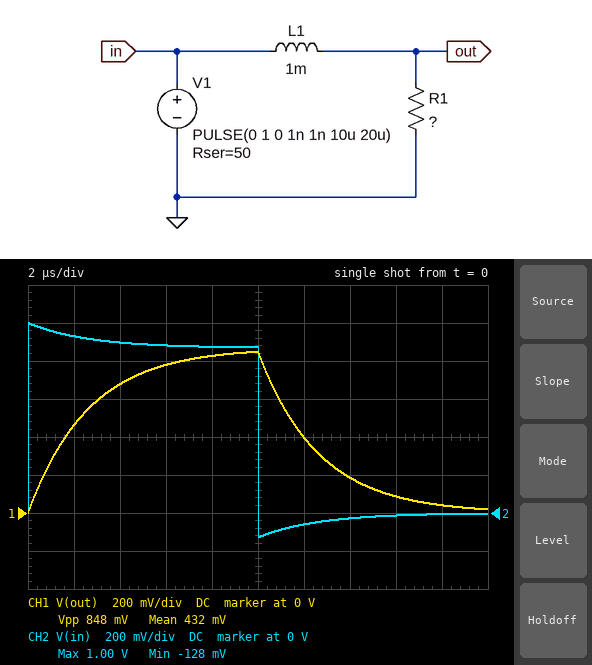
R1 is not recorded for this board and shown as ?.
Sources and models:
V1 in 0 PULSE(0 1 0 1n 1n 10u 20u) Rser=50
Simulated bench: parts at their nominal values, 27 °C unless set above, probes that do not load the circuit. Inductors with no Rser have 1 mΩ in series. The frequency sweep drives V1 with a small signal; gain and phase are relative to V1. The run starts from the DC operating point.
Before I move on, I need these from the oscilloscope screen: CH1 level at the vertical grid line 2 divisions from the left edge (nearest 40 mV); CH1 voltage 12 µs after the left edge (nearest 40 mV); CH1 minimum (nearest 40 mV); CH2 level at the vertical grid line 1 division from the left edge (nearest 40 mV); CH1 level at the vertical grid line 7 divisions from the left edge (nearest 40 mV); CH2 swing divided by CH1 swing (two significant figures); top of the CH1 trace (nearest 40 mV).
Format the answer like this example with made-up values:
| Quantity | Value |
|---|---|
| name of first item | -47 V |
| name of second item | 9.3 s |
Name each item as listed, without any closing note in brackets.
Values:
| Quantity | Value |
|---|---|
| CH1 level at the vertical grid line 2 divisions from the left edge | 680 mV |
| CH1 voltage 12 µs after the left edge | 400 mV |
| CH1 minimum | 0 V |
| CH2 level at the vertical grid line 1 division from the left edge | 920 mV |
| CH1 level at the vertical grid line 7 divisions from the left edge | 200 mV |
| CH2 swing divided by CH1 swing | 1.3 |
| top of the CH1 trace | 840 mV |
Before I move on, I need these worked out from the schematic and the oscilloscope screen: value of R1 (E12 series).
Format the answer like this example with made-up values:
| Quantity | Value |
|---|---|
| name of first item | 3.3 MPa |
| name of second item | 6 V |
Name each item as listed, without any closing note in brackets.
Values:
| Quantity | Value |
|---|---|
| value of R1 | 330 Ω |
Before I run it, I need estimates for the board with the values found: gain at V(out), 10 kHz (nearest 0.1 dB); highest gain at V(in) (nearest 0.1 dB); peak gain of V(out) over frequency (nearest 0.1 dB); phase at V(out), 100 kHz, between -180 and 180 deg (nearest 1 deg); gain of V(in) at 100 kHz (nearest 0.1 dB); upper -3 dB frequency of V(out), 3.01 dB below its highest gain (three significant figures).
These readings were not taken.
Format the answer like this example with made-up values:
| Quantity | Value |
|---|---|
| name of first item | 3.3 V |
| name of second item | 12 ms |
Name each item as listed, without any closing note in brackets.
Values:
| Quantity | Value |
|---|---|
| gain at V(out), 10 kHz | -1.3 dB |
| highest gain at V(in) | 0 dB |
| peak gain of V(out) over frequency | -1.2 dB |
| phase at V(out), 100 kHz, between -180 and 180 deg | -59 deg |
| gain of V(in) at 100 kHz | -0.3 dB |
| upper -3 dB frequency of V(out), 3.01 dB below its highest gain | 60.5 kHz |
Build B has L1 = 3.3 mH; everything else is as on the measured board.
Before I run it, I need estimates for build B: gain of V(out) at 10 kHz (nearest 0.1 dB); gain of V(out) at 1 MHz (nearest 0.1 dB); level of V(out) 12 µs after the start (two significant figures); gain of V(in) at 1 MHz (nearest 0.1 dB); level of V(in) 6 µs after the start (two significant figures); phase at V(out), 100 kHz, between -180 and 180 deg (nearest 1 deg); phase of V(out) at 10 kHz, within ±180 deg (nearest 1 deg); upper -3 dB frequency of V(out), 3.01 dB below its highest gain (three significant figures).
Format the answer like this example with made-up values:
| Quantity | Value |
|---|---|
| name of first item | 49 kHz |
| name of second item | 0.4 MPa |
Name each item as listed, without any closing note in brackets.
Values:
| Quantity | Value |
|---|---|
| gain of V(out) at 10 kHz | -2.4 dB |
| gain of V(out) at 1 MHz | -36.0 dB |
| level of V(out) 12 µs after the start | 470 mV |
| gain of V(in) at 1 MHz | 0 dB |
| level of V(in) 6 µs after the start | 930 mV |
| phase at V(out), 100 kHz, between -180 and 180 deg | -80 deg |
| phase of V(out) at 10 kHz, within ±180 deg | -29 deg |
| upper -3 dB frequency of V(out), 3.01 dB below its highest gain | 18.3 kHz |
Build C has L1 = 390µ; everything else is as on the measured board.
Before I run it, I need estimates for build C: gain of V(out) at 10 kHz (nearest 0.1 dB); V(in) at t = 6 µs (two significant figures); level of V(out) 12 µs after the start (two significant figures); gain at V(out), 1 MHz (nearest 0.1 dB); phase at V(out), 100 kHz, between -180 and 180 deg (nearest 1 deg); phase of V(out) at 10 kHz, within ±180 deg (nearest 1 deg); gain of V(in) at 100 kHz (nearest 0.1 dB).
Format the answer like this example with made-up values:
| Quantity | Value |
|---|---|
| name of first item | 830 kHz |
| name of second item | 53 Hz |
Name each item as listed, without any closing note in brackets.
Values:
| Quantity | Value |
|---|---|
| gain of V(out) at 10 kHz | -1.2 dB |
| V(in) at t = 6 µs | 870 mV |
| level of V(out) 12 µs after the start | 120 mV |
| gain at V(out), 1 MHz | -17.5 dB |
| phase at V(out), 100 kHz, between -180 and 180 deg | -33 deg |
| phase of V(out) at 10 kHz, within ±180 deg | -4 deg |
| gain of V(in) at 100 kHz | -0.8 dB |
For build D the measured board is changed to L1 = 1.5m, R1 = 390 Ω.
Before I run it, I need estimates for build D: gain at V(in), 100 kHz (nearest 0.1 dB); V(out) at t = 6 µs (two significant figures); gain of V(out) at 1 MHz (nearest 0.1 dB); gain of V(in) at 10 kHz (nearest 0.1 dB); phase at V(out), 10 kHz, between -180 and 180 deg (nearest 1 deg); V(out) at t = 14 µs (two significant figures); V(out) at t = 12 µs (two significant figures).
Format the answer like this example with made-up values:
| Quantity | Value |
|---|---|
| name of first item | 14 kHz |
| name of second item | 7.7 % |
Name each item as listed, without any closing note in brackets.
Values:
| Quantity | Value |
|---|---|
| gain at V(in), 100 kHz | -0.2 dB |
| V(out) at t = 6 µs | 730 mV |
| gain of V(out) at 1 MHz | -27.7 dB |
| gain of V(in) at 10 kHz | -1.0 dB |
| phase at V(out), 10 kHz, between -180 and 180 deg | -12 deg |
| V(out) at t = 14 µs | 260 mV |
| V(out) at t = 12 µs | 470 mV |
